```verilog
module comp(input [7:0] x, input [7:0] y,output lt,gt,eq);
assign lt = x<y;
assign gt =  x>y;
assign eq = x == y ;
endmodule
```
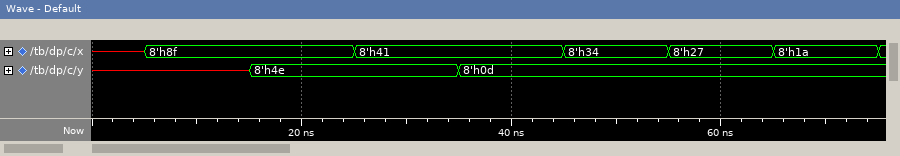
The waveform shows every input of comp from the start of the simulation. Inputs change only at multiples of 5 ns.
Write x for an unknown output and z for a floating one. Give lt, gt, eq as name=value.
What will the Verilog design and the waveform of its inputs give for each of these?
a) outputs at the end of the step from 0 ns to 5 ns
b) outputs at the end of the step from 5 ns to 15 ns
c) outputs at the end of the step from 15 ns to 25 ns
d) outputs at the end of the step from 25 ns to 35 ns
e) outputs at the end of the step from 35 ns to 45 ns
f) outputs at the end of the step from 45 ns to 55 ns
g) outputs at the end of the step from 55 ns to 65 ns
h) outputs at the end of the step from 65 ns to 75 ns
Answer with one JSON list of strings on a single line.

["lt=x, gt=x, eq=x", "lt=x, gt=x, eq=x", "lt=0, gt=1, eq=0", "lt=1, gt=0, eq=0", "lt=0, gt=1, eq=0", "lt=0, gt=1, eq=0", "lt=0, gt=1, eq=0", "lt=0, gt=1, eq=0"]
